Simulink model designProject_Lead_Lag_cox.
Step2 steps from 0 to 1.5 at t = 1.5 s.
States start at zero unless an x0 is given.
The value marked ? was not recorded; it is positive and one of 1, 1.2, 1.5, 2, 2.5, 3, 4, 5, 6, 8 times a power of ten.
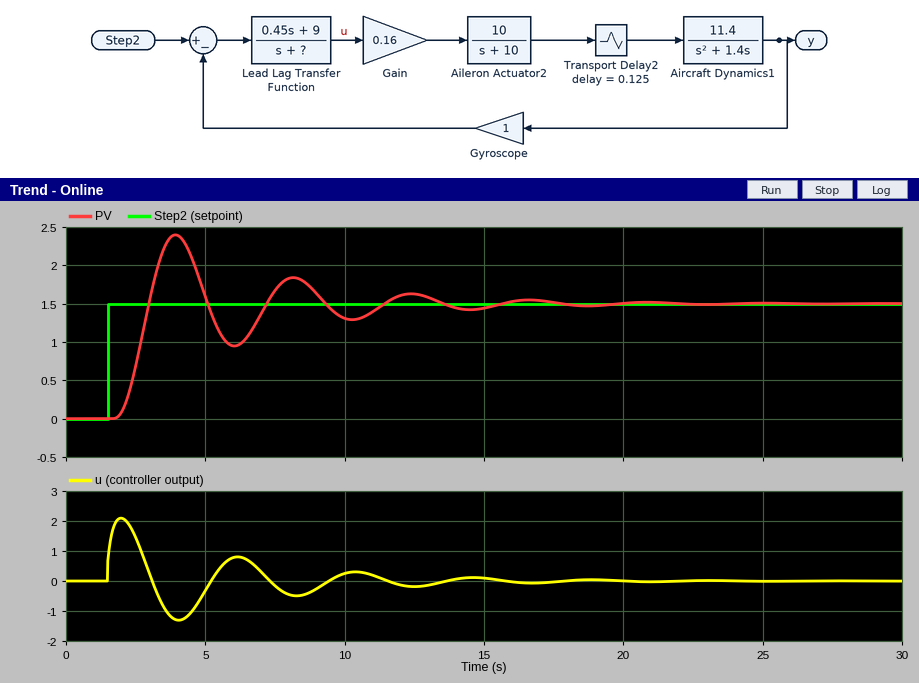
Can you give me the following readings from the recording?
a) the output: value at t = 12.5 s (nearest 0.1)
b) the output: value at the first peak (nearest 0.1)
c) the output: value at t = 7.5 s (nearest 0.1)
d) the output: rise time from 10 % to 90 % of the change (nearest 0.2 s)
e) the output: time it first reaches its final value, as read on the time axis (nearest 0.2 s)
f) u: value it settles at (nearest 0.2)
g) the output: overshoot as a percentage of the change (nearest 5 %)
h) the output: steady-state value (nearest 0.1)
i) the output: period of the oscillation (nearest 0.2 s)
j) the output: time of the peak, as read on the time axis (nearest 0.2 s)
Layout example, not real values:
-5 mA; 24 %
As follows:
1.6; 2.4; 1.7; 0.8 s; 3.0 s; 0.0; 60 %; 1.5; 4.2 s; 4.0 s
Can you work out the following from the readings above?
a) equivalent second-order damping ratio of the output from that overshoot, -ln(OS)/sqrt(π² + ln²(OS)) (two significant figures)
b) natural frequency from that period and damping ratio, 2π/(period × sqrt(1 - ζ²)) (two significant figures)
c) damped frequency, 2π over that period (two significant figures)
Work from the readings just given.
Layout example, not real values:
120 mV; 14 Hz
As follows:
0.16; 1.5 rad/s; 1.5 rad/s
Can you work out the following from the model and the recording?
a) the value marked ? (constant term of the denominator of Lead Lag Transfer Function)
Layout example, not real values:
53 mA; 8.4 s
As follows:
6
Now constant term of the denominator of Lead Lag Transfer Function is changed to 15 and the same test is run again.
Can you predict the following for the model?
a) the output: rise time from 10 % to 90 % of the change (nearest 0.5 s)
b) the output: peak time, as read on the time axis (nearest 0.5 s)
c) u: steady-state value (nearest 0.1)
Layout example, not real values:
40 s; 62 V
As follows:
1.5 s; 5.5 s; 0.0
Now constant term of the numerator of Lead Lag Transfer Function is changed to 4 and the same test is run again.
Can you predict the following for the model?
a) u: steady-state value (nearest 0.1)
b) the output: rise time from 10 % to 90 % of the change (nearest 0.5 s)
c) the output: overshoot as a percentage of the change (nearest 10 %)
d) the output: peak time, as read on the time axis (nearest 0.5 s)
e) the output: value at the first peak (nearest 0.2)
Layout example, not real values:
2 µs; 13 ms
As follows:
0.0; 1.5 s; 20 %; 5.0 s; 1.8
